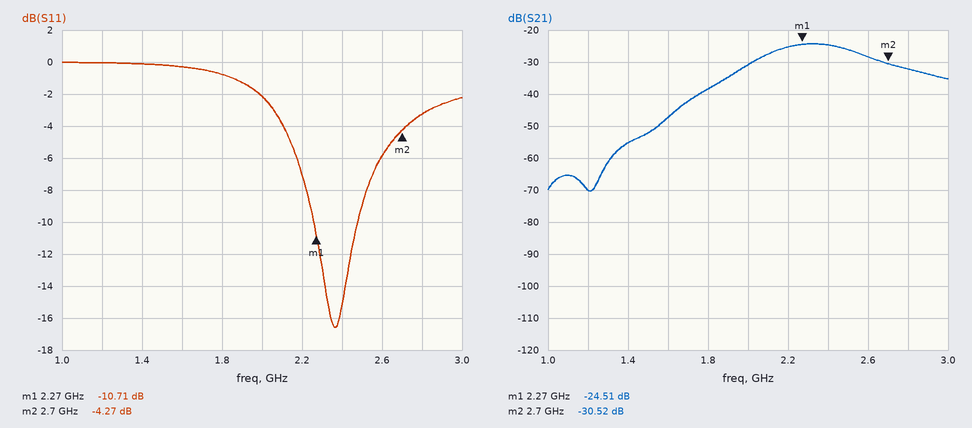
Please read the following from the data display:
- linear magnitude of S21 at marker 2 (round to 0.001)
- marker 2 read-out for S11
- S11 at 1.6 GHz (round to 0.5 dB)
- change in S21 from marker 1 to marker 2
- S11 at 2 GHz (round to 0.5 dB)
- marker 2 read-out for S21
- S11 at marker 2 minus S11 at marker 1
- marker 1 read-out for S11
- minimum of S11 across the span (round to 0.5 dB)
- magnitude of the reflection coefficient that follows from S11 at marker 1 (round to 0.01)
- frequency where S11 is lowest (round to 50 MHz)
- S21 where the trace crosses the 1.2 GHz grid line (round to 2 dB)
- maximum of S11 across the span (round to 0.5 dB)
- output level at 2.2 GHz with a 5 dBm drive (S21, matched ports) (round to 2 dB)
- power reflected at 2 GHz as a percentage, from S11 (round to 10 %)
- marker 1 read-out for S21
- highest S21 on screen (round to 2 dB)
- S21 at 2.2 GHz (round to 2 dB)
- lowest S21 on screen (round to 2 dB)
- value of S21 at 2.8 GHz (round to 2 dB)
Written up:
0.030
-4.27 dB
-0.5 dB
-6.01 dB
-2.0 dB
-30.52 dB
6.44 dB
-10.71 dB
-16.5 dB
0.29
2.35 GHz
-70 dB
0.0 dB
-20 dBm
60 %
-24.51 dB
-24 dB
-26 dB
-70 dB
-32 dB
